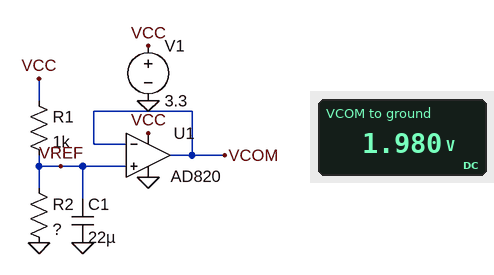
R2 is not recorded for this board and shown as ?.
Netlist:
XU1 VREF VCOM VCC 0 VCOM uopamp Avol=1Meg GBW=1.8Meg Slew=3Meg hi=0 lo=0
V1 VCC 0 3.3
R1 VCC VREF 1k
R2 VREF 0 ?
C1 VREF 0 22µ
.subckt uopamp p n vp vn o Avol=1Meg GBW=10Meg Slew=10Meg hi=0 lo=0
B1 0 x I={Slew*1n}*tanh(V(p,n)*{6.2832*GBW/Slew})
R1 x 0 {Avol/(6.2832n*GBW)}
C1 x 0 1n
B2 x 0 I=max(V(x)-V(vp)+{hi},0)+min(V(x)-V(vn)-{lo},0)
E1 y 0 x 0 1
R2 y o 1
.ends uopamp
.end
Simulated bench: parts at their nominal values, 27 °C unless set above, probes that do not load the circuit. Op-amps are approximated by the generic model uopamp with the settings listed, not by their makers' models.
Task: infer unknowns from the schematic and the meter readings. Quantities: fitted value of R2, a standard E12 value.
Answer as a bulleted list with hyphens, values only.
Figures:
- 1.5 kΩ
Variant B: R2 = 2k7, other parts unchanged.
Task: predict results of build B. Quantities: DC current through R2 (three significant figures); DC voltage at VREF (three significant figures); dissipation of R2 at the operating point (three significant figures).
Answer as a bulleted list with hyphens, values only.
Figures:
- 892 µA
- 2.41 V
- 2.15 mW
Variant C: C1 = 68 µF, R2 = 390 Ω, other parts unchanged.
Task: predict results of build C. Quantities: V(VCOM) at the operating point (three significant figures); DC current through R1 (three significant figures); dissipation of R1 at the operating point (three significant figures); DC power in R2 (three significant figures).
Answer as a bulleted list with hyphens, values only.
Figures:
- 926 mV
- 2.37 mA
- 5.64 mW
- 2.20 mW
